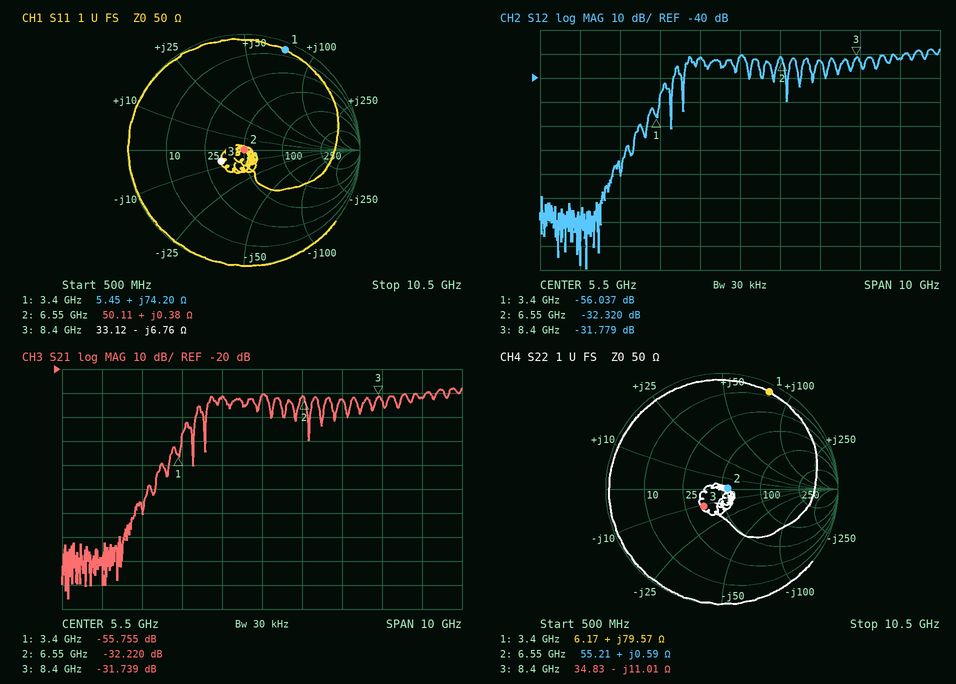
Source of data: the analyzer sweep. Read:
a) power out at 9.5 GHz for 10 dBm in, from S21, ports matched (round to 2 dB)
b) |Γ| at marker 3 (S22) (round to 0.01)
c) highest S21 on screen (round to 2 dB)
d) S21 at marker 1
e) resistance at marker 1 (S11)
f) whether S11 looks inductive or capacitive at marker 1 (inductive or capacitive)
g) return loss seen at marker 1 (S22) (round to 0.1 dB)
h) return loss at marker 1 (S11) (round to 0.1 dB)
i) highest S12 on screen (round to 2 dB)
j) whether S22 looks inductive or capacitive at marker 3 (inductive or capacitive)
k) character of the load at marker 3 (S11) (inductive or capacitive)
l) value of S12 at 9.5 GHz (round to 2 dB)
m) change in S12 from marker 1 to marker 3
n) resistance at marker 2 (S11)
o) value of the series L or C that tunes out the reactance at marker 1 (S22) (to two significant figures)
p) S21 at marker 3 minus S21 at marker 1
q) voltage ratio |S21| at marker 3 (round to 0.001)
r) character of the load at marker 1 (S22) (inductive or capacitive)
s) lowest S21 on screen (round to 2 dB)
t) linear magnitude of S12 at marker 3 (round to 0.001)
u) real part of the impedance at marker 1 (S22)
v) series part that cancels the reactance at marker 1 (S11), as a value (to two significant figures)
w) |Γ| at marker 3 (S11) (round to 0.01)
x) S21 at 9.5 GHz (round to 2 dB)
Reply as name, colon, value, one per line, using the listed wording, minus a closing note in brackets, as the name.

power out at 9.5 GHz for 10 dBm in, from S21, ports matched: -22 dBm
|Γ| at marker 3 (S22): 0.22
highest S21 on screen: -28 dB
S21 at marker 1: -55.755 dB
resistance at marker 1: 5.45 Ω
whether S11 looks inductive or capacitive at marker 1: inductive
return loss seen at marker 1 (S22): 0.6 dB
return loss at marker 1 (S11): 0.6 dB
highest S12 on screen: -28 dB
whether S22 looks inductive or capacitive at marker 3: capacitive
character of the load at marker 3 (S11): capacitive
value of S12 at 9.5 GHz: -32 dB
change in S12 from marker 1 to marker 3: 24.258 dB
resistance at marker 2: 50.11 Ω
value of the series L or C that tunes out the reactance at marker 1 (S22): 590 fF
S21 at marker 3 minus S21 at marker 1: 24.016 dB
voltage ratio |S21| at marker 3: 0.026
character of the load at marker 1 (S22): inductive
lowest S21 on screen: -116 dB
linear magnitude of S12 at marker 3: 0.026
real part of the impedance at marker 1: 6.17 Ω
series part that cancels the reactance at marker 1 (S11), as a value: 630 fF
|Γ| at marker 3 (S11): 0.22
S21 at 9.5 GHz: -32 dB
